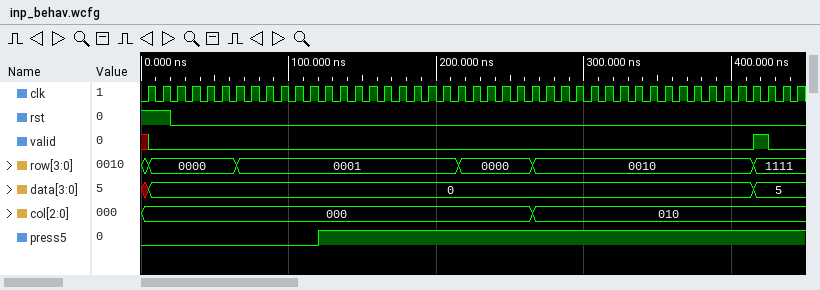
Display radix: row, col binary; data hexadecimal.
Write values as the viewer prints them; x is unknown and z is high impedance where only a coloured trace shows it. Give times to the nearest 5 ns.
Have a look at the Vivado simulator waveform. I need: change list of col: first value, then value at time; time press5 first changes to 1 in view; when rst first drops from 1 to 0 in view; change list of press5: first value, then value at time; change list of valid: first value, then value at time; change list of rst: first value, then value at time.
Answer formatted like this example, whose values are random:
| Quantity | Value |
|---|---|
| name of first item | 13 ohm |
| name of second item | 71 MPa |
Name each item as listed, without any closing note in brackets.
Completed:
| Quantity | Value |
|---|---|
| change list of col: first value, then value at time | 000, 010 at 265 ns |
| time press5 first changes to 1 in view | 120 ns |
| when rst first drops from 1 to 0 in view | 20 ns |
| change list of press5: first value, then value at time | 0, 1 at 120 ns |
| change list of valid: first value, then value at time | x, 0 at 5 ns, 1 at 415 ns, 0 at 425 ns |
| change list of rst: first value, then value at time | 1, 0 at 20 ns |
